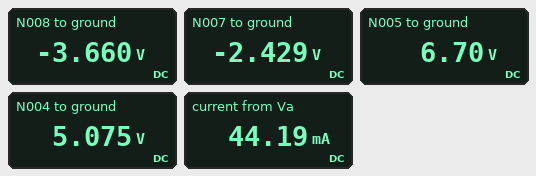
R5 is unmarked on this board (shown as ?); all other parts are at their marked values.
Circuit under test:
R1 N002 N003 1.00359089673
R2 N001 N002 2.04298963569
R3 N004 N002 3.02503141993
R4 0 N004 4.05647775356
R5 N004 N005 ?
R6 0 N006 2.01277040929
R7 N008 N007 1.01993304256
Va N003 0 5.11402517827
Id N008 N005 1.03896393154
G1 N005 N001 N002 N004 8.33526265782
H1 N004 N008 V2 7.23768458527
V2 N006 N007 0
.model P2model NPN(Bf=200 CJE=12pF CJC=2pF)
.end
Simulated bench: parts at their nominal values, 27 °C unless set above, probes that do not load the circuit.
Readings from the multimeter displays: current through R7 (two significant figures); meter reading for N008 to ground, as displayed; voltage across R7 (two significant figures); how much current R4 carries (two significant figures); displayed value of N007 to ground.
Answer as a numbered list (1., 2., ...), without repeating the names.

1. 1.2 A
2. -3.660 V
3. 1.2 V
4. 1.3 A
5. -2.429 V
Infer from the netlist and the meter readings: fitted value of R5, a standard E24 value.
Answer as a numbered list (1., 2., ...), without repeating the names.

1. 1.5 Ω
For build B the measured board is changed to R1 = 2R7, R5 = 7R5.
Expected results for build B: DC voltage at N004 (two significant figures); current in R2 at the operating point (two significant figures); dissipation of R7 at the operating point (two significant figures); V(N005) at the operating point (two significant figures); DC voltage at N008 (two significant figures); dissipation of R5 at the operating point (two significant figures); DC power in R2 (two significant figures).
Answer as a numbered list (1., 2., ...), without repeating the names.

1. 5.0 V
2. 45 mA
3. 1.4 W
4. 13 V
5. -3.6 V
6. 8.8 W
7. 4.2 mW
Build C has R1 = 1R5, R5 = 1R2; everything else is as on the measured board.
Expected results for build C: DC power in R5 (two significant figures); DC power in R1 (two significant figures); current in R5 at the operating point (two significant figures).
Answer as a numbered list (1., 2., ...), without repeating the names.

1. 1.4 W
2. 2.9 mW
3. 1.1 A
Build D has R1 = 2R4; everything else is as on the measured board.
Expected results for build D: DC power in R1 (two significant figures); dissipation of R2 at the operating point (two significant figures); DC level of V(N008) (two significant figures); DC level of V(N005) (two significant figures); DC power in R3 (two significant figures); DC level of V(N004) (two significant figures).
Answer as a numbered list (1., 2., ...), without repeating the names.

1. 4.6 mW
2. 4.2 mW
3. -3.6 V
4. 6.6 V
5. 9.8 µW
6. 5.0 V
